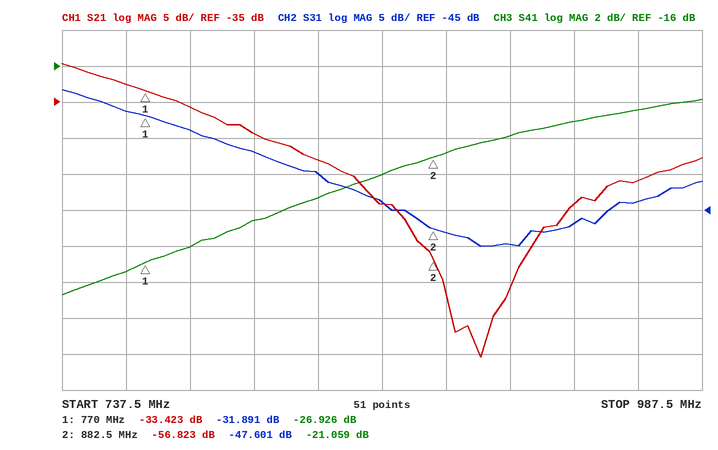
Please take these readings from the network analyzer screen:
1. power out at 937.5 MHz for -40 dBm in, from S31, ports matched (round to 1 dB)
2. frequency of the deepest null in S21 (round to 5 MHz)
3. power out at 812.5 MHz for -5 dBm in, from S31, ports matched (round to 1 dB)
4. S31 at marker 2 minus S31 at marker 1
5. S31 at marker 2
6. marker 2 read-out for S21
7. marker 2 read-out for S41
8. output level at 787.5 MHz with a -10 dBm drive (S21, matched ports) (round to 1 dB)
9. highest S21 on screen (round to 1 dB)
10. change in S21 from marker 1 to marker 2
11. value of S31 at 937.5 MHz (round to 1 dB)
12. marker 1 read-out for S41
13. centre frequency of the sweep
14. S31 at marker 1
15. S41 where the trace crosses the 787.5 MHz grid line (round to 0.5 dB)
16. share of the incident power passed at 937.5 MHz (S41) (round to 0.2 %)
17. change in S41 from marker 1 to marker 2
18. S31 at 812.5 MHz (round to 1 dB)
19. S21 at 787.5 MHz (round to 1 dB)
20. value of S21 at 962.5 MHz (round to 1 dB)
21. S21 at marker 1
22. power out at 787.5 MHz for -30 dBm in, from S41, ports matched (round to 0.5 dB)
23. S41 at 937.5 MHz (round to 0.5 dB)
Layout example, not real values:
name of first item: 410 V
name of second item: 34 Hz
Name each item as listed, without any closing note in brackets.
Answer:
power out at 937.5 MHz for -40 dBm in, from S31, ports matched: -87 dBm
frequency of the deepest null in S21: 900 MHz
power out at 812.5 MHz for -5 dBm in, from S31, ports matched: -42 dBm
S31 at marker 2 minus S31 at marker 1: -15.710 dB
S31 at marker 2: -47.601 dB
marker 2 read-out for S21: -56.823 dB
marker 2 read-out for S41: -21.059 dB
output level at 787.5 MHz with a -10 dBm drive (S21, matched ports): -46 dBm
highest S21 on screen: -30 dB
change in S21 from marker 1 to marker 2: -23.400 dB
value of S31 at 937.5 MHz: -47 dB
marker 1 read-out for S41: -26.926 dB
centre frequency of the sweep: 862.5 MHz
S31 at marker 1: -31.891 dB
S41 where the trace crosses the 787.5 MHz grid line: -26.0 dB
share of the incident power passed at 937.5 MHz (S41): 1.2 %
change in S41 from marker 1 to marker 2: 5.867 dB
S31 at 812.5 MHz: -37 dB
S21 at 787.5 MHz: -36 dB
value of S21 at 962.5 MHz: -46 dB
S21 at marker 1: -33.423 dB
power out at 787.5 MHz for -30 dBm in, from S41, ports matched: -56.0 dBm
S41 at 937.5 MHz: -19.0 dB
